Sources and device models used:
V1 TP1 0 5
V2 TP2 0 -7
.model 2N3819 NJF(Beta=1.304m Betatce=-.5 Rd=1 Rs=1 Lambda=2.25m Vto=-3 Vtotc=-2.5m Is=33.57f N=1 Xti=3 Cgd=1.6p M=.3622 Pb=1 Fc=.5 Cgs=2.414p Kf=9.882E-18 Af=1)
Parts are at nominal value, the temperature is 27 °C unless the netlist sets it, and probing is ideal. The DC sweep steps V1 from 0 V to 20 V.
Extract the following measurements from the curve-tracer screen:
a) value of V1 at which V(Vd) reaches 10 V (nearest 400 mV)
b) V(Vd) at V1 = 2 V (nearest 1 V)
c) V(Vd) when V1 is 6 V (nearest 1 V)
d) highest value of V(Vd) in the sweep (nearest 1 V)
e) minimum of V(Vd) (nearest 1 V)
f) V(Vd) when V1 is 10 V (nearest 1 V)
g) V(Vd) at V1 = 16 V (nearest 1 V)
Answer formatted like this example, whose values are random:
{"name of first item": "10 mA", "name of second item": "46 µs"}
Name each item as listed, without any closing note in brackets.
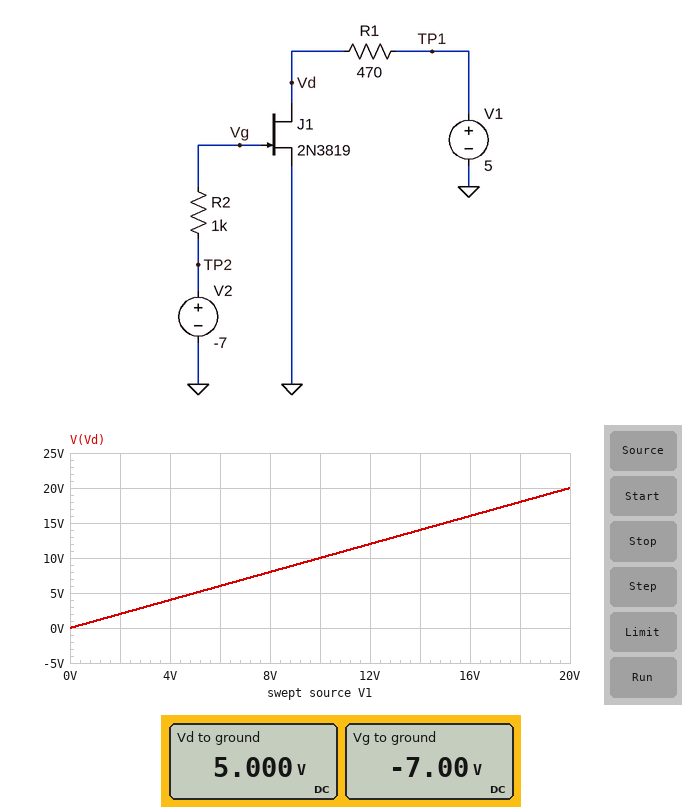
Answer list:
{"value of V1 at which V(Vd) reaches 10 V": "10.0 V", "V(Vd) at V1 = 2 V": "2 V", "V(Vd) when V1 is 6 V": "6 V", "highest value of V(Vd) in the sweep": "20 V", "minimum of V(Vd)": "0 V", "V(Vd) when V1 is 10 V": "10 V", "V(Vd) at V1 = 16 V": "16 V"}
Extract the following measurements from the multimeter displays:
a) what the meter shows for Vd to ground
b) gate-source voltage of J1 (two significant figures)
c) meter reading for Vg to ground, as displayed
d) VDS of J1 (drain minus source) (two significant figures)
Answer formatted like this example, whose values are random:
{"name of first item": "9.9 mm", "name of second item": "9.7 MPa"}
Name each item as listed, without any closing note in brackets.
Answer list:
{"what the meter shows for Vd to ground": "5.000 V", "gate-source voltage of J1": "-7.0 V", "meter reading for Vg to ground, as displayed": "-7.00 V", "VDS of J1 (drain minus source)": "5.0 V"}
